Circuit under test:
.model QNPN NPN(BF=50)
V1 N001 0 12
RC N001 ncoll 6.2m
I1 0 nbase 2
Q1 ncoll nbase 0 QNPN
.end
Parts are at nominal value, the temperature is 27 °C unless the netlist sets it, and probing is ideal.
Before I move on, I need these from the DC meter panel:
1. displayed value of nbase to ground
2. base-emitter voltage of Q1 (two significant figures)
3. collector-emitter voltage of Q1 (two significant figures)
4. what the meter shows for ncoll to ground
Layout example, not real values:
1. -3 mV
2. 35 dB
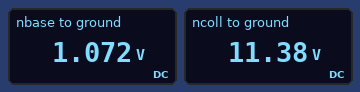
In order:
1. 1.072 V
2. 1.1 V
3. 11 V
4. 11.38 V
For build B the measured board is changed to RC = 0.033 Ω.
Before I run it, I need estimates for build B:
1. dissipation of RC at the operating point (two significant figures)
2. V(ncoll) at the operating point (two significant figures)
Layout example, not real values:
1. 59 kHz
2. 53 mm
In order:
1. 330 W
2. 8.7 V
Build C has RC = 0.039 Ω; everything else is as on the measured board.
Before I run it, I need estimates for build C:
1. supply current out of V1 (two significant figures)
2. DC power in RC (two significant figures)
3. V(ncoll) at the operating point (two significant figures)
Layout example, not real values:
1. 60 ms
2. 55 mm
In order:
1. 100 A
2. 390 W
3. 8.1 V
